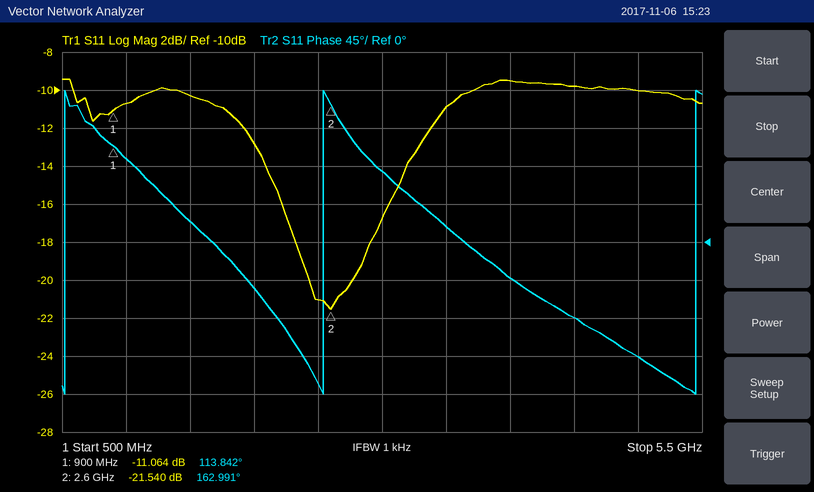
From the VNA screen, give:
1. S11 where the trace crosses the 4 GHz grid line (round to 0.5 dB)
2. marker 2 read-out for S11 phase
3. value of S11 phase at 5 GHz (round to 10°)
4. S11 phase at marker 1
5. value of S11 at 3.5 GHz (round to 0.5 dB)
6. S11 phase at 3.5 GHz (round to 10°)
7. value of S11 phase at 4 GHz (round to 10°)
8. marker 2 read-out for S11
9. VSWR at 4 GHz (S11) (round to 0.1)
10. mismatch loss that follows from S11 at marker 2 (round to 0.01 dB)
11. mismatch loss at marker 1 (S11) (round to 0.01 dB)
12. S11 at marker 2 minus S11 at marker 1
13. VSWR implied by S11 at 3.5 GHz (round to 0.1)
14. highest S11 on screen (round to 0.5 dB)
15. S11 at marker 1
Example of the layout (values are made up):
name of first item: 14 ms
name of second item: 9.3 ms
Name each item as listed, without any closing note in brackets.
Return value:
S11 where the trace crosses the 4 GHz grid line: -9.5 dB
marker 2 read-out for S11 phase: 162.991°
value of S11 phase at 5 GHz: -140°
S11 phase at marker 1: 113.842°
value of S11 at 3.5 GHz: -11.0 dB
S11 phase at 3.5 GHz: 20°
value of S11 phase at 4 GHz: -40°
marker 2 read-out for S11: -21.540 dB
VSWR at 4 GHz (S11): 2.0
mismatch loss that follows from S11 at marker 2: 0.03 dB
mismatch loss at marker 1 (S11): 0.35 dB
S11 at marker 2 minus S11 at marker 1: -10.476 dB
VSWR implied by S11 at 3.5 GHz: 1.8
highest S11 on screen: -9.5 dB
S11 at marker 1: -11.064 dB
